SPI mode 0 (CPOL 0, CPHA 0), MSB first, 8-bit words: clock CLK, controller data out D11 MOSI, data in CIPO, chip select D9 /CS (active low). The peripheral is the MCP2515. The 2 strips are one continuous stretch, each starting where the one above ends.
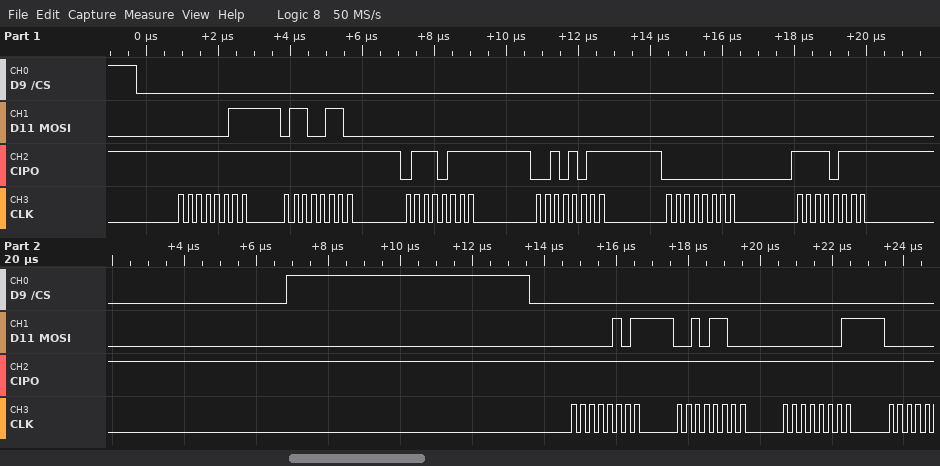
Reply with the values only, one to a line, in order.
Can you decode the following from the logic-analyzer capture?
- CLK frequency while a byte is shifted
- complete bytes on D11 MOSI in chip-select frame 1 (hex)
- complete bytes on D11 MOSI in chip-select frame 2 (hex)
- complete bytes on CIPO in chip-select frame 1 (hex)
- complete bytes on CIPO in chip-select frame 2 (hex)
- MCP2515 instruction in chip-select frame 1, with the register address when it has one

4 MHz
0x03 0x66 0x00 0x00 0x00 0x00
0x05 0x2C 0x01
0xFF 0xFF 0x77 0x2B 0x00 0xF7
0xFF 0xFF 0xFF
READ 0x66
